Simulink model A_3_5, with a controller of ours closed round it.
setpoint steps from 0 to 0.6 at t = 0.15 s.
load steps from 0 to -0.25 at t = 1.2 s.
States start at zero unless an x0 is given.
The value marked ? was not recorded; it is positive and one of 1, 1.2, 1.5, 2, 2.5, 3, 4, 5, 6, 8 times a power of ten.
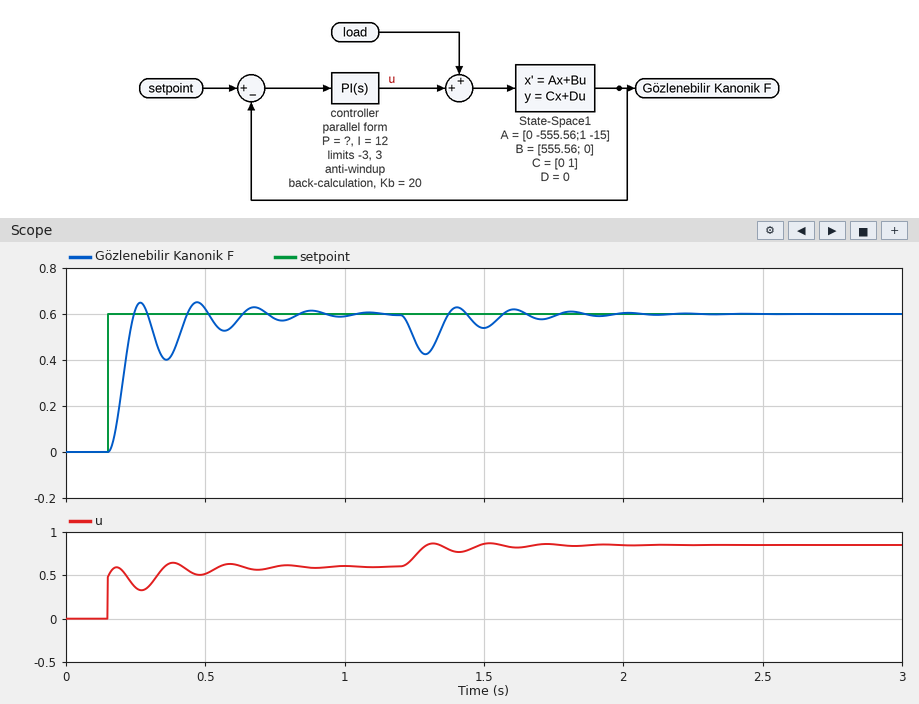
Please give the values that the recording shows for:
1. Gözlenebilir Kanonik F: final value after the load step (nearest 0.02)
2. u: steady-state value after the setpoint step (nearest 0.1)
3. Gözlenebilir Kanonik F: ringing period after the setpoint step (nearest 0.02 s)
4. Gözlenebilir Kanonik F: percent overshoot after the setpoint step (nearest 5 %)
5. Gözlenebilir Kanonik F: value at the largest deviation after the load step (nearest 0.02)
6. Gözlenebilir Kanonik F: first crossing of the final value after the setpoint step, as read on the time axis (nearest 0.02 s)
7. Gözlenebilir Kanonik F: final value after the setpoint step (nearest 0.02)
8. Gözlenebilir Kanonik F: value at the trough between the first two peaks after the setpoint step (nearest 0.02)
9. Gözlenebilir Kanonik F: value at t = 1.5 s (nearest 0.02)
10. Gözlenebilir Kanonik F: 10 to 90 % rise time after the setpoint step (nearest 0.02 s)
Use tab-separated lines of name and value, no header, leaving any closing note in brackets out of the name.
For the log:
Gözlenebilir Kanonik F: final value after the load step	0.60
u: steady-state value after the setpoint step	0.6
Gözlenebilir Kanonik F: ringing period after the setpoint step	0.20 s
Gözlenebilir Kanonik F: percent overshoot after the setpoint step	10 %
Gözlenebilir Kanonik F: value at the largest deviation after the load step	0.42
Gözlenebilir Kanonik F: first crossing of the final value after the setpoint step, as read on the time axis	0.24 s
Gözlenebilir Kanonik F: final value after the setpoint step	0.60
Gözlenebilir Kanonik F: value at the trough between the first two peaks after the setpoint step	0.40
Gözlenebilir Kanonik F: value at t = 1.5 s	0.54
Gözlenebilir Kanonik F: 10 to 90 % rise time after the setpoint step	0.06 s
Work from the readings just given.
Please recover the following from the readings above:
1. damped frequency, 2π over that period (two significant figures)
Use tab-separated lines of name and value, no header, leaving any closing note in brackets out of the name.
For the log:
damped frequency, 2π over that period	31 rad/s
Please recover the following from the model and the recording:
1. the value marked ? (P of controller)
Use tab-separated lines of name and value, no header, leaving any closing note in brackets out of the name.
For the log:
the value marked ?	0.8
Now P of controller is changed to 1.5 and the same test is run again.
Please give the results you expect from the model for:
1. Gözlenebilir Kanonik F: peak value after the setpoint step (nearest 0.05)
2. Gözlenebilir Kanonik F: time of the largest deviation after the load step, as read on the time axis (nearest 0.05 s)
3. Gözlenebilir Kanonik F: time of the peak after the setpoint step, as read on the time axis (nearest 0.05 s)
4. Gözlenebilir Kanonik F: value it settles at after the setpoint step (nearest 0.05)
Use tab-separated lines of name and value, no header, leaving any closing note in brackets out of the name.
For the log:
Gözlenebilir Kanonik F: peak value after the setpoint step	0.70
Gözlenebilir Kanonik F: time of the largest deviation after the load step, as read on the time axis	1.30 s
Gözlenebilir Kanonik F: time of the peak after the setpoint step, as read on the time axis	0.25 s
Gözlenebilir Kanonik F: value it settles at after the setpoint step	0.60
